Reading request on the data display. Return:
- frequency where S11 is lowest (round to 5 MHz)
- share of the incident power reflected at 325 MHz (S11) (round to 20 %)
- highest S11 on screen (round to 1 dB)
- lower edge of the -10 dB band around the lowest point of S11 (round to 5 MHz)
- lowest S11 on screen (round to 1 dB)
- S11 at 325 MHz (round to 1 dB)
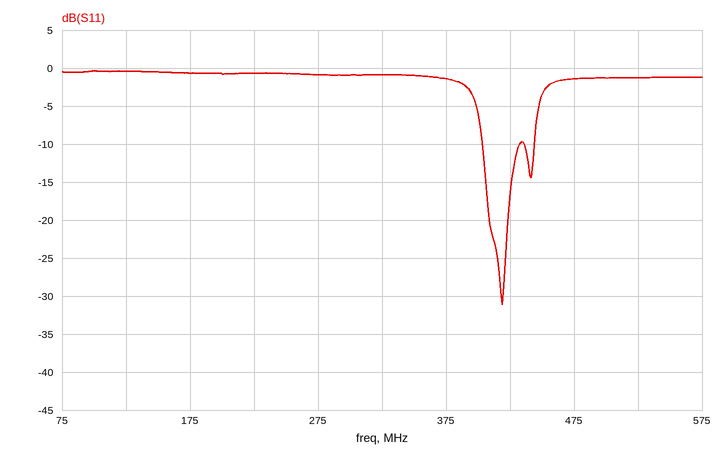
420 MHz
80 %
0 dB
405 MHz
-31 dB
-1 dB
